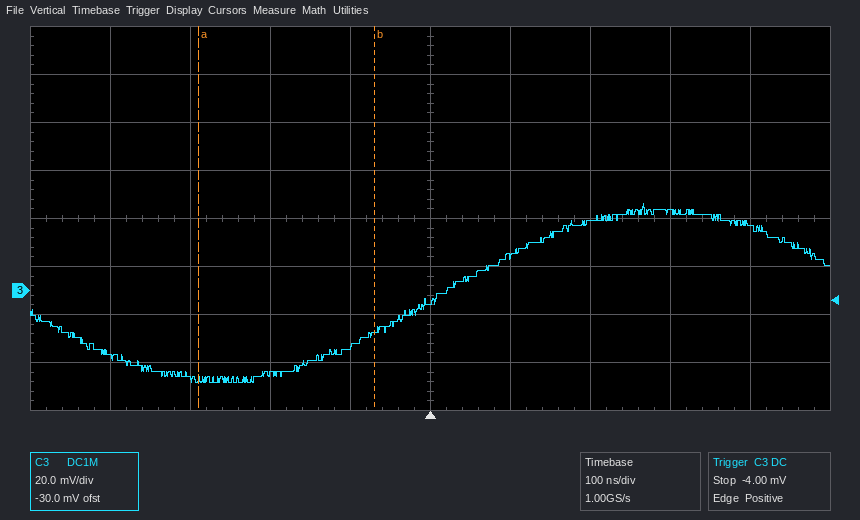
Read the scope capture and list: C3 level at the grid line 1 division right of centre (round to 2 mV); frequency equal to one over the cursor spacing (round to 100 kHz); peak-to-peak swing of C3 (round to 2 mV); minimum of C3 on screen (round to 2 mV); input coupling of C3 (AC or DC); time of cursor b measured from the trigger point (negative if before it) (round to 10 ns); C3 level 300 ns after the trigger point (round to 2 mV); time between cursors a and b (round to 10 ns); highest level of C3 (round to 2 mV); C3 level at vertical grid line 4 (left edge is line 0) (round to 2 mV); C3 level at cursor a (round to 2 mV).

14 mV
4.5 MHz
74 mV
-38 mV
DC
-70 ns
32 mV
220 ns
36 mV
-24 mV
-38 mV
